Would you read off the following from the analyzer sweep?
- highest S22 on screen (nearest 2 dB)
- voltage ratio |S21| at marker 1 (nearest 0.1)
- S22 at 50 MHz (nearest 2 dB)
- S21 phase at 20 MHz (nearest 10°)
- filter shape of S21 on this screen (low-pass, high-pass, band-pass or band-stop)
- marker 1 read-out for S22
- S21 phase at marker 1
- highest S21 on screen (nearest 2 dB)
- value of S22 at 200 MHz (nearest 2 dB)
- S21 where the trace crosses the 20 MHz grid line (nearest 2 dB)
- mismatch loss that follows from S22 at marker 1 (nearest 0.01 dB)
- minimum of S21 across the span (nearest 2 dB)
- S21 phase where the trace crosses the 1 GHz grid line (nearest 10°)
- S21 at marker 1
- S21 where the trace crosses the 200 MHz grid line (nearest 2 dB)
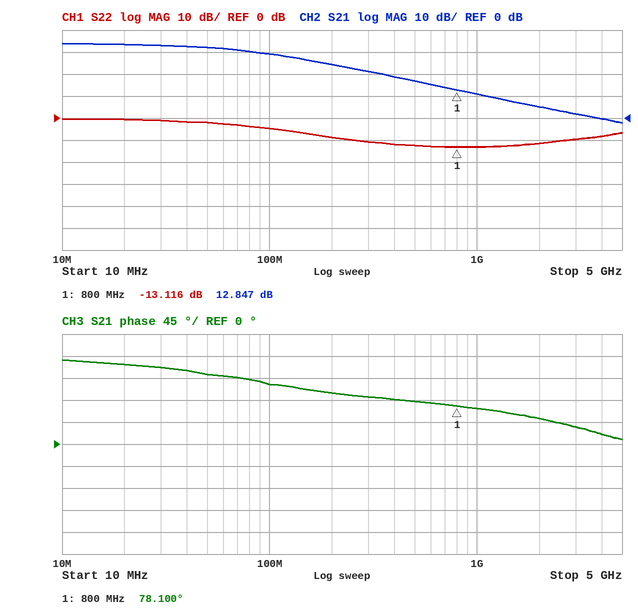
0 dB
4.4
-2 dB
160°
low-pass
-13.116 dB
78.100°
34 dB
-8 dB
34 dB
0.22 dB
-2 dB
70°
12.847 dB
24 dB
